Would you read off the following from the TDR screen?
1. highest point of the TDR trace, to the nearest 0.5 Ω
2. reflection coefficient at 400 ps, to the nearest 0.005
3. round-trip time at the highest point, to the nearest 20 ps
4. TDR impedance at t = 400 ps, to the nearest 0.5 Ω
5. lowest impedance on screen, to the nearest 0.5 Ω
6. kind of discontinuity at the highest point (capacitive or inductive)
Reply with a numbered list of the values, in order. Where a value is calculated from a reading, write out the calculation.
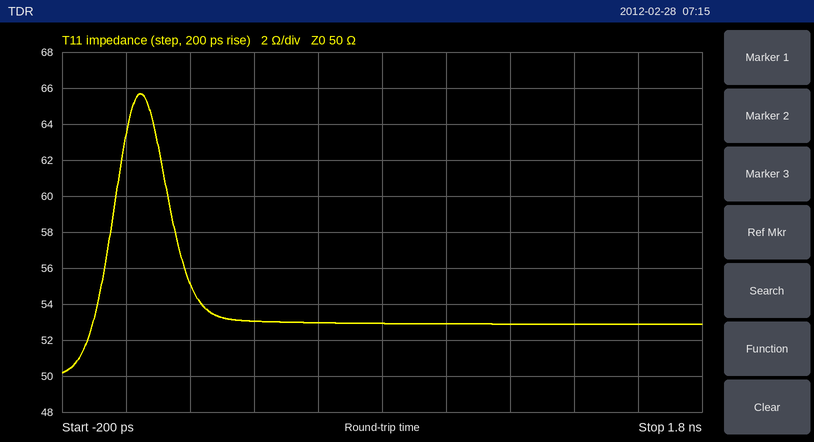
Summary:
1. 65.5 Ω
2. (53 − 50)/(53 + 50) ≈ +0.0291, so +0.030 to the nearest 0.005
3. 40 ps
4. 53.0 Ω
5. 50.0 Ω
6. inductive
